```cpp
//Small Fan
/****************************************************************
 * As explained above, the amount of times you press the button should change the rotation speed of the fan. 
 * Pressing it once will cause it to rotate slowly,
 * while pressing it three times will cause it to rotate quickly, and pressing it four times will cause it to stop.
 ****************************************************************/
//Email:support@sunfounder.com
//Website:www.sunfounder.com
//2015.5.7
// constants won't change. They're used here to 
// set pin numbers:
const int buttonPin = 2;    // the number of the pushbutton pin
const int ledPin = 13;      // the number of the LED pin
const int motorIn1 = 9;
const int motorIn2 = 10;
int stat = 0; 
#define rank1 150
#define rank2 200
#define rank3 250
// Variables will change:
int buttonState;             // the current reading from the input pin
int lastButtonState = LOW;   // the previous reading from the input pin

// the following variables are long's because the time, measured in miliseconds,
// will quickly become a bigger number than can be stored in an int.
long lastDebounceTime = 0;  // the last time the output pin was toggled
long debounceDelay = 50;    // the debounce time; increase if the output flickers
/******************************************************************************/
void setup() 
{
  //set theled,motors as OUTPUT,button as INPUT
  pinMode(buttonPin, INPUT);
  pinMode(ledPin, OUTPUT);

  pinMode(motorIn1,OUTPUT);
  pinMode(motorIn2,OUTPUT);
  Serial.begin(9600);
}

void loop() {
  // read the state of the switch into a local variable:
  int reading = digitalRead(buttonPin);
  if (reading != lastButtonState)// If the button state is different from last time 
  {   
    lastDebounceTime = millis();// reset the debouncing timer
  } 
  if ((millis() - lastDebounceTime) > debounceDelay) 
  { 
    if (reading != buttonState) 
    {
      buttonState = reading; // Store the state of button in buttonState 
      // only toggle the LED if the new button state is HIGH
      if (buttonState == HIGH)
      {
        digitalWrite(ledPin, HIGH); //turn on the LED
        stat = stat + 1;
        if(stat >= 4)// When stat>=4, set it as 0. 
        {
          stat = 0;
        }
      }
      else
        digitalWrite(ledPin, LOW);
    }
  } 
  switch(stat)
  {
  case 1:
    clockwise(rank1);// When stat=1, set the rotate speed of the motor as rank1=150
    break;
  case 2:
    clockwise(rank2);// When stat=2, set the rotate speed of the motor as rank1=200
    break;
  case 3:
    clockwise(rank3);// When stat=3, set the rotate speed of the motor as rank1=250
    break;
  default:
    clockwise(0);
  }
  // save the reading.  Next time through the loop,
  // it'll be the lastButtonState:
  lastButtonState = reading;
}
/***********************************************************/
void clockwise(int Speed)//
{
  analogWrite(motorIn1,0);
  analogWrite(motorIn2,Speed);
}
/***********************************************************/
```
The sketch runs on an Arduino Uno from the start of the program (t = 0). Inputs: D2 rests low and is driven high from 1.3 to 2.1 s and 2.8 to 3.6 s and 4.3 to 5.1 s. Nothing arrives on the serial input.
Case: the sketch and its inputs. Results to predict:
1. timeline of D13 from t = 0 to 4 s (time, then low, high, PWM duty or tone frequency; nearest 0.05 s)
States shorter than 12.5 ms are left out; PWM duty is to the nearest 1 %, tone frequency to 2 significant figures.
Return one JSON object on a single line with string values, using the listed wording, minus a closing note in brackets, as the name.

{"timeline of D13 from t = 0 to 4 s": "0 s low; 1.35 s high; 2.15 s low; 2.85 s high; 3.65 s low"}
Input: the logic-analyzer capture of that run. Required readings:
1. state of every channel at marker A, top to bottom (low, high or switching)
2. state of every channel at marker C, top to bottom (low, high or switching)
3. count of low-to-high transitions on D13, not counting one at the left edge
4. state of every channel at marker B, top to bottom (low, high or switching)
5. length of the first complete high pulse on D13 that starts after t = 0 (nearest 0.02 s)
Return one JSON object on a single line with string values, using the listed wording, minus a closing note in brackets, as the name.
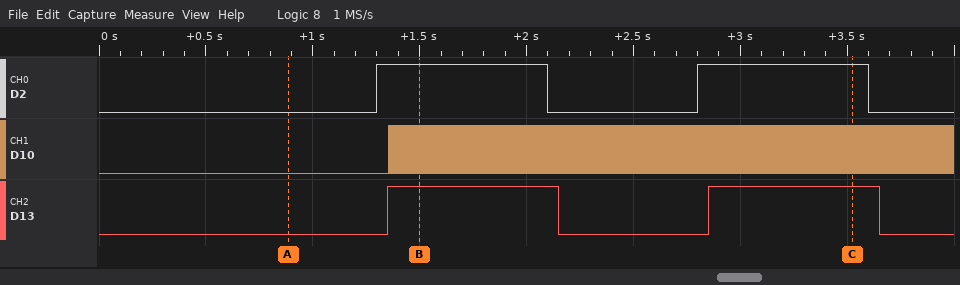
{"state of every channel at marker A, top to bottom": "D2 low, D10 low, D13 low", "state of every channel at marker C, top to bottom": "D2 high, D10 switching, D13 high", "count of low-to-high transitions on D13, not counting one at the left edge": "2", "state of every channel at marker B, top to bottom": "D2 high, D10 switching, D13 high", "length of the first complete high pulse on D13 that starts after t = 0": "0.80 s"}
